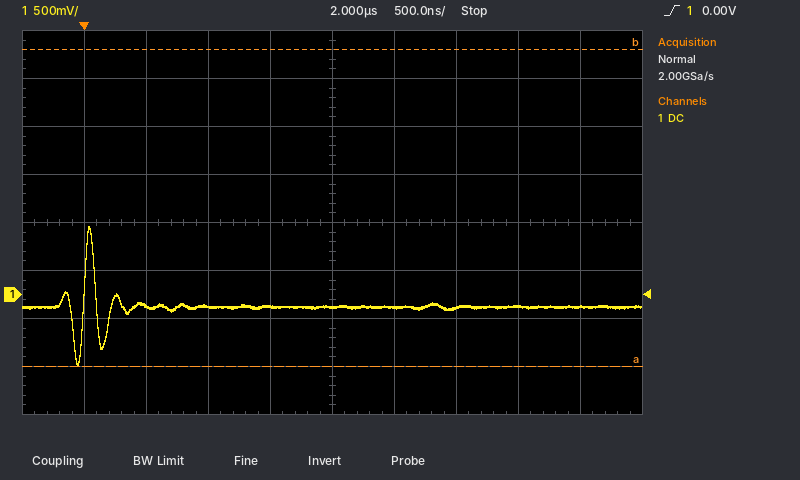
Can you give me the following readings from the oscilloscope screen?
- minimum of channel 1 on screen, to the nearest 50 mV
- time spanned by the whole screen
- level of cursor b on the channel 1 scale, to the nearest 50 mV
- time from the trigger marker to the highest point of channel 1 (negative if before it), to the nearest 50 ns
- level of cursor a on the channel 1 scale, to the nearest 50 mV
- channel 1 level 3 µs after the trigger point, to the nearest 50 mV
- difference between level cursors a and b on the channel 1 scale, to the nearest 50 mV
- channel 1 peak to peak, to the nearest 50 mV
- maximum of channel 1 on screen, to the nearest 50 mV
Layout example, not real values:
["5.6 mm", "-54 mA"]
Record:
["-750 mV", "5 µs", "2.55 V", "+50 ns", "-750 mV", "-150 mV", "3.30 V", "1.45 V", "700 mV"]
